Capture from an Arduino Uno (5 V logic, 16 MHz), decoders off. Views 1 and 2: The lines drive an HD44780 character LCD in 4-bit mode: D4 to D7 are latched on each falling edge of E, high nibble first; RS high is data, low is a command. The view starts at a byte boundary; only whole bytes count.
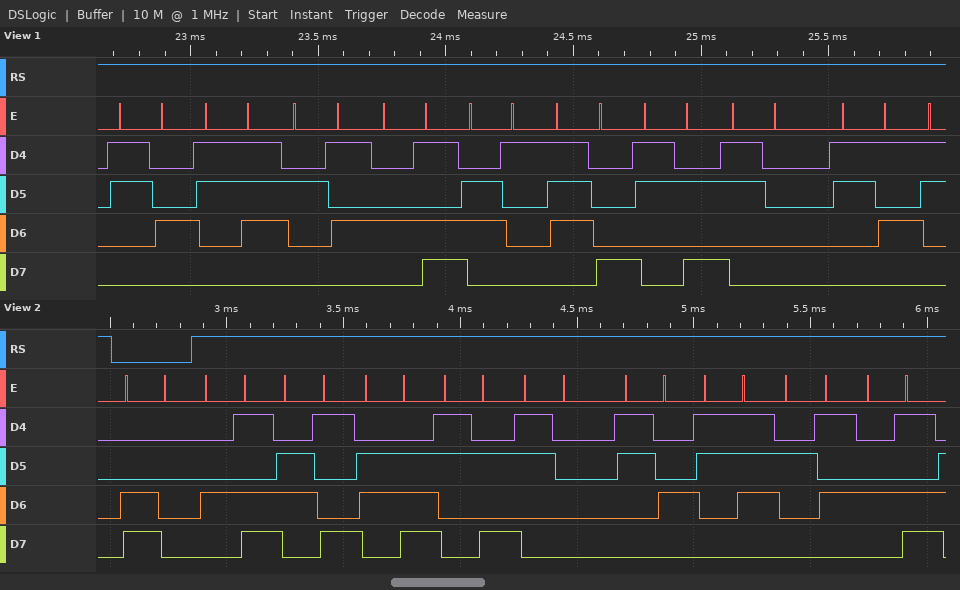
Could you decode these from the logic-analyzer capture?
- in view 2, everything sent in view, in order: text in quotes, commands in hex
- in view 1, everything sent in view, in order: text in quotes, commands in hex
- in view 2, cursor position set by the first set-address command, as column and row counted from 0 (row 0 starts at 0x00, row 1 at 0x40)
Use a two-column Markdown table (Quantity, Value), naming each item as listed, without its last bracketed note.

| Quantity | Value |
|---|---|
| in view 2, everything sent in view, in order: text in quotes, commands in hex | 0xC0 "Min:047%M" |
| in view 1, everything sent in view, in order: text in quotes, commands in hex | "47%Max:05" |
| in view 2, cursor position set by the first set-address command, as column and row counted from 0 | column 0, row 1 |
